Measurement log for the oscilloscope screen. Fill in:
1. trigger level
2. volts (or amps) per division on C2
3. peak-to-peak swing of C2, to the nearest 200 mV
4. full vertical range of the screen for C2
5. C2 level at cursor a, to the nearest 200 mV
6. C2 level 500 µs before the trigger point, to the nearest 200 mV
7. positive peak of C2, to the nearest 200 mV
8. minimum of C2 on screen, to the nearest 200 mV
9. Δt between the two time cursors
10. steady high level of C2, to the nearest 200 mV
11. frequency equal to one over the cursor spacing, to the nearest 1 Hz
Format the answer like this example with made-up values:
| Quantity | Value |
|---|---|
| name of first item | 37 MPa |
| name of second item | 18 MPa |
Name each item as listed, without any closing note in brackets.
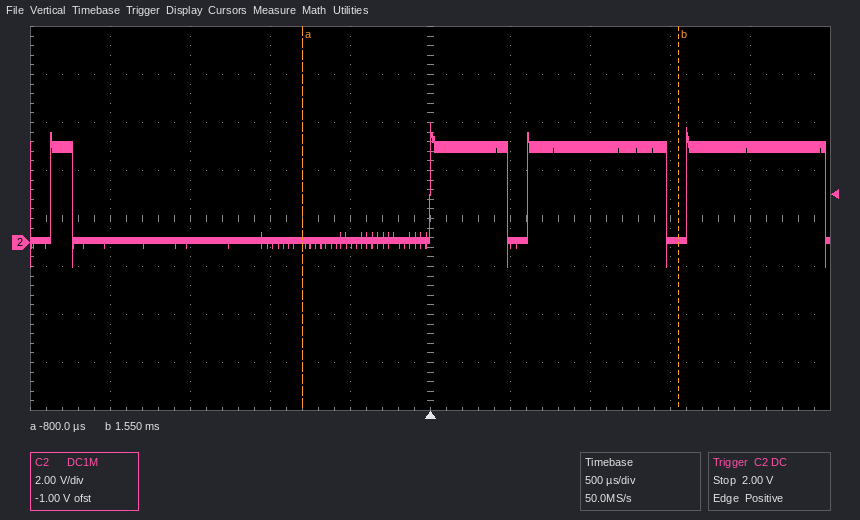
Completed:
| Quantity | Value |
|---|---|
| trigger level | 2.00 V |
| volts (or amps) per division on C2 | 2 V |
| peak-to-peak swing of C2, to the nearest 200 mV | 6.0 V |
| full vertical range of the screen for C2 | 16 V |
| C2 level at cursor a, to the nearest 200 mV | 0.0 V |
| C2 level 500 µs before the trigger point, to the nearest 200 mV | 0.0 V |
| positive peak of C2, to the nearest 200 mV | 5.0 V |
| minimum of C2 on screen, to the nearest 200 mV | -1.0 V |
| Δt between the two time cursors | 2.35 ms |
| steady high level of C2, to the nearest 200 mV | 4.0 V |
| frequency equal to one over the cursor spacing, to the nearest 1 Hz | 426 Hz |
